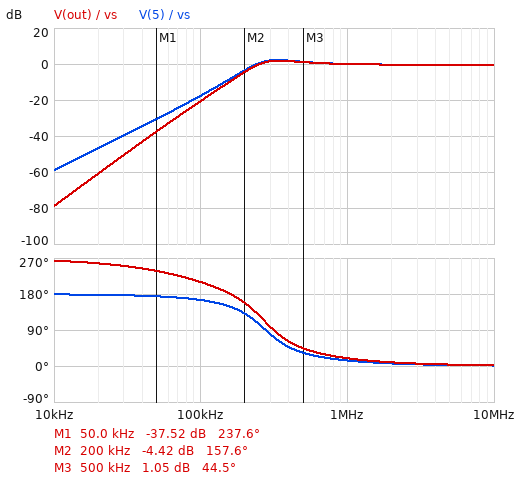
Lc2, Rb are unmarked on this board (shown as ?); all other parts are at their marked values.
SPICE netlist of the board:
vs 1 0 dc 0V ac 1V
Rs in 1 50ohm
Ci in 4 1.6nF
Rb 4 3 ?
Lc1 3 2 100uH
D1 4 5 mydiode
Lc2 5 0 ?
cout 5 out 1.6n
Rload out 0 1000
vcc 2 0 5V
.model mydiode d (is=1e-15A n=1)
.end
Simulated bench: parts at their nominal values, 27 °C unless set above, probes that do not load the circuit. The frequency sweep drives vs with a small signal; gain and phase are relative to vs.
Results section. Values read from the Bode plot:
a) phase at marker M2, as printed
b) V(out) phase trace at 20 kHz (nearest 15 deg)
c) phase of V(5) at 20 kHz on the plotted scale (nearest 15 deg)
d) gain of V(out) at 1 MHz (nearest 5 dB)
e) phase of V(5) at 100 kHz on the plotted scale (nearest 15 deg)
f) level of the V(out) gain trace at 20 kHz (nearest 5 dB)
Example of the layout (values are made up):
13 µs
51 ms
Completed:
157.6 deg
255 deg
180 deg
0 dB
165 deg
-60 dB
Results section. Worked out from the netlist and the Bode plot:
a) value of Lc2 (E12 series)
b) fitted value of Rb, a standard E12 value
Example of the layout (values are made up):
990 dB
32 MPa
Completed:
180 µH
1 kΩ
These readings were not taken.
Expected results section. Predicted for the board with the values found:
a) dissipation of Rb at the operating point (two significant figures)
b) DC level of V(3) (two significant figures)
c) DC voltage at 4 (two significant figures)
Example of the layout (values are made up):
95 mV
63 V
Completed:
18 mW
5.0 V
750 mV
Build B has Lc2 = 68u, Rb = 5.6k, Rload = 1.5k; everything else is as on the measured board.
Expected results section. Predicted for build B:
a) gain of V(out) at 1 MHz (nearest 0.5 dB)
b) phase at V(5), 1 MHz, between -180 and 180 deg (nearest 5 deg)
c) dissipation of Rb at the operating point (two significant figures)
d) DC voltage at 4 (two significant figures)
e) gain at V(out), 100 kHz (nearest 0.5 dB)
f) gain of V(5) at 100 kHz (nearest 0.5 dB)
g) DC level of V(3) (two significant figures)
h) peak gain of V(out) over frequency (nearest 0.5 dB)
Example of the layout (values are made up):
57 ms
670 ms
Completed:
1.0 dB
20 deg
3.3 mW
710 mV
-28.5 dB
-27.0 dB
5.0 V
5.0 dB
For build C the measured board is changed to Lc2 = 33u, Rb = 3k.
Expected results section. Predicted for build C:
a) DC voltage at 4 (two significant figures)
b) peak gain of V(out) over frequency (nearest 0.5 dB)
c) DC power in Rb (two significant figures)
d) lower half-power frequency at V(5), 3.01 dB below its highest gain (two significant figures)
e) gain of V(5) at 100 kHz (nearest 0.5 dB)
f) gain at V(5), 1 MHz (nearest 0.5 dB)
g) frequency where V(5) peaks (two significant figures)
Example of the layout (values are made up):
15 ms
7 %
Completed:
720 mV
3.5 dB
6.1 mW
560 kHz
-33.5 dB
2.5 dB
740 kHz
